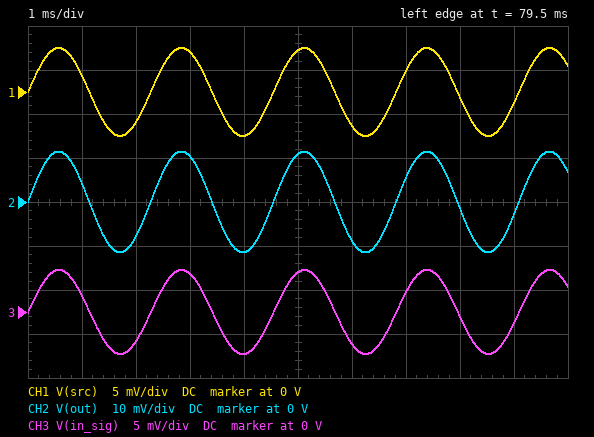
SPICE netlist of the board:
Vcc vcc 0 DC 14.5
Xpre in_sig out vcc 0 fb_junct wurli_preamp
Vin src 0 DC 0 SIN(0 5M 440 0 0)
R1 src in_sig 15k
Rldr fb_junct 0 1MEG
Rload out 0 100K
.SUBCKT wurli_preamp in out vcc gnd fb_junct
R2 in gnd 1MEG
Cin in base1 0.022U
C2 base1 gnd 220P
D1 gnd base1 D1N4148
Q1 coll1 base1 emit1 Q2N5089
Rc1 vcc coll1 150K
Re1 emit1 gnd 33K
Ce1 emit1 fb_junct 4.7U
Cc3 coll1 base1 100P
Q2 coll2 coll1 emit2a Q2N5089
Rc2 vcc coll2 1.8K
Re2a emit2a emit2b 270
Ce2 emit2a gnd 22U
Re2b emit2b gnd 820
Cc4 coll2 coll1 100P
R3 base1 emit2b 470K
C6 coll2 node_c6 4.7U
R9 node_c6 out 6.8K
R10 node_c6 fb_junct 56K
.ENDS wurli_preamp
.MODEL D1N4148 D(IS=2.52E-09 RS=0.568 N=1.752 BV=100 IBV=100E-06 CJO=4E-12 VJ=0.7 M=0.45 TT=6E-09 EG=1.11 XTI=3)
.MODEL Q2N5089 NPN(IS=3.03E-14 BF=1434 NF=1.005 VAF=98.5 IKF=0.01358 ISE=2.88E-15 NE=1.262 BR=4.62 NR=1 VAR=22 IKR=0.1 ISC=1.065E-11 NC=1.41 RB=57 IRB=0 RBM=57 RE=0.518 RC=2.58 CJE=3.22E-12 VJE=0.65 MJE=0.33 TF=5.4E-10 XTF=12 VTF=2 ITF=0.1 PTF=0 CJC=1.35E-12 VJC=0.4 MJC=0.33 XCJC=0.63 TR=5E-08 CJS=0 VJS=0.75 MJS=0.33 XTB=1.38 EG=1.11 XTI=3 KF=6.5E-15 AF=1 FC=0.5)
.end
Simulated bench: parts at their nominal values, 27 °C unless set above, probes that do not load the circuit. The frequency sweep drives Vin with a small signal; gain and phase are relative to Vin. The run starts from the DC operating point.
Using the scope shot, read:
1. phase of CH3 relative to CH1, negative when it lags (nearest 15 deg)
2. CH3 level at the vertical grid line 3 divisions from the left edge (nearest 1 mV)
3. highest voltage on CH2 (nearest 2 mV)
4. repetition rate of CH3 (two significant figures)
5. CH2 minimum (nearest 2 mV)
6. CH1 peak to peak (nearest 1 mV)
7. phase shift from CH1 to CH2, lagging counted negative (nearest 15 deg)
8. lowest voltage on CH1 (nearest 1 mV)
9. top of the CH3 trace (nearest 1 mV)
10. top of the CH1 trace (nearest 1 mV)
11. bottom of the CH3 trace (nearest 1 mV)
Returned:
0 deg
4 mV
12 mV
440 Hz
-12 mV
10 mV
0 deg
-5 mV
5 mV
5 mV
-5 mV
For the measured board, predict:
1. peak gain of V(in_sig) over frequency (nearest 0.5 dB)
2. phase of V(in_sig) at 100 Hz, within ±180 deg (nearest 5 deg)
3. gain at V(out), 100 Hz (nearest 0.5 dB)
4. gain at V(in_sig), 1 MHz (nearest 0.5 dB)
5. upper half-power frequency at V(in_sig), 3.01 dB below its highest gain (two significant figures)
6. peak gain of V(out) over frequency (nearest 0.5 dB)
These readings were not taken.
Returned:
0 dB
0 deg
7.0 dB
-29.5 dB
33 kHz
7.0 dB
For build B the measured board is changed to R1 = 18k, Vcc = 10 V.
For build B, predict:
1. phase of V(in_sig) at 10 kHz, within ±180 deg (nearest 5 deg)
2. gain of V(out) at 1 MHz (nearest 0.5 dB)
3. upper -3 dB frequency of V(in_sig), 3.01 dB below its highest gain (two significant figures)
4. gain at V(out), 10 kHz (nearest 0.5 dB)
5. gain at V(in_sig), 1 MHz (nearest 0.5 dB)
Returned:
-20 deg
-32.0 dB
27 kHz
6.0 dB
-31.0 dB
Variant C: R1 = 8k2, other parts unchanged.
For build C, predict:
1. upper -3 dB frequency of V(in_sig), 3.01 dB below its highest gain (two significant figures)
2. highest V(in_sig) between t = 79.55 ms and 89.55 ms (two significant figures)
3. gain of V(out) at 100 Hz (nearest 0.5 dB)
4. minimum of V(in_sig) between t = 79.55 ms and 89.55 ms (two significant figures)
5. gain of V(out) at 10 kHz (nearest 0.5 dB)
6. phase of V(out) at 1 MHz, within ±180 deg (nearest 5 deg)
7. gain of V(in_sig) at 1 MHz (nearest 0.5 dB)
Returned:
60 kHz
4.9 mV
7.5 dB
-4.9 mV
7.0 dB
100 deg
-24.5 dB
